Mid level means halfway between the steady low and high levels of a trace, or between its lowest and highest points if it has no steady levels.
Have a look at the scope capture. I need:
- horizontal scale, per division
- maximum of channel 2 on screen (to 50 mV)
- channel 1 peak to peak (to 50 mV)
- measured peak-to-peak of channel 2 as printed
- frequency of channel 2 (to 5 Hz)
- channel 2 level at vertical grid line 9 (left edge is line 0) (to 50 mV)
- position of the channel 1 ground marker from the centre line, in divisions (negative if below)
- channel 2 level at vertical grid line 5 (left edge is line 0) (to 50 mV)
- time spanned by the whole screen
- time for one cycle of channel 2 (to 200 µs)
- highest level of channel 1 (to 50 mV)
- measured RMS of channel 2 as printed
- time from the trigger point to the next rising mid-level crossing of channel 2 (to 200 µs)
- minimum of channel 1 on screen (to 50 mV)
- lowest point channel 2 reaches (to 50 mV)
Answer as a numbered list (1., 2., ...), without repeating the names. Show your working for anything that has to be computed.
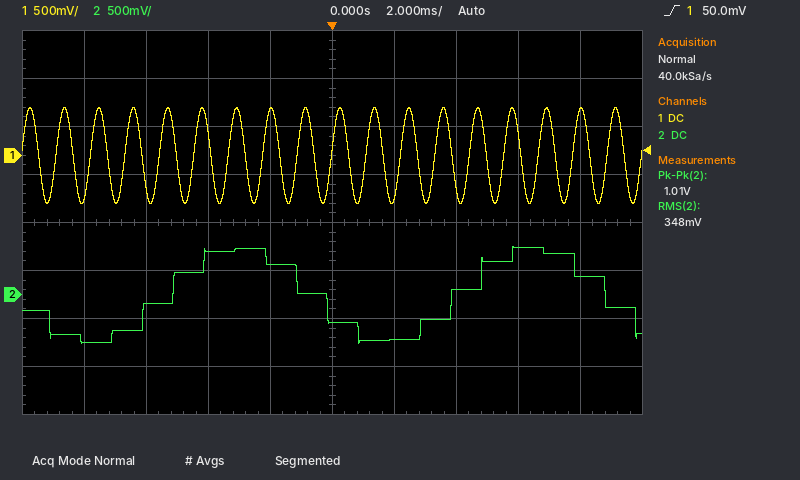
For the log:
1. 2 ms
2. 500 mV
3. 500 mV − (-500 mV) = 1.00 V
4. 1.01 V
5. 1 / 9.0 ms ≈ 111 Hz, so 110 Hz to the nearest 5 Hz
6. 200 mV
7. +1.4 div
8. -300 mV
9. 20 ms
10. 9.0 ms
11. 500 mV
12. 348 mV
13. 3.8 ms
14. -500 mV
15. -500 mV
